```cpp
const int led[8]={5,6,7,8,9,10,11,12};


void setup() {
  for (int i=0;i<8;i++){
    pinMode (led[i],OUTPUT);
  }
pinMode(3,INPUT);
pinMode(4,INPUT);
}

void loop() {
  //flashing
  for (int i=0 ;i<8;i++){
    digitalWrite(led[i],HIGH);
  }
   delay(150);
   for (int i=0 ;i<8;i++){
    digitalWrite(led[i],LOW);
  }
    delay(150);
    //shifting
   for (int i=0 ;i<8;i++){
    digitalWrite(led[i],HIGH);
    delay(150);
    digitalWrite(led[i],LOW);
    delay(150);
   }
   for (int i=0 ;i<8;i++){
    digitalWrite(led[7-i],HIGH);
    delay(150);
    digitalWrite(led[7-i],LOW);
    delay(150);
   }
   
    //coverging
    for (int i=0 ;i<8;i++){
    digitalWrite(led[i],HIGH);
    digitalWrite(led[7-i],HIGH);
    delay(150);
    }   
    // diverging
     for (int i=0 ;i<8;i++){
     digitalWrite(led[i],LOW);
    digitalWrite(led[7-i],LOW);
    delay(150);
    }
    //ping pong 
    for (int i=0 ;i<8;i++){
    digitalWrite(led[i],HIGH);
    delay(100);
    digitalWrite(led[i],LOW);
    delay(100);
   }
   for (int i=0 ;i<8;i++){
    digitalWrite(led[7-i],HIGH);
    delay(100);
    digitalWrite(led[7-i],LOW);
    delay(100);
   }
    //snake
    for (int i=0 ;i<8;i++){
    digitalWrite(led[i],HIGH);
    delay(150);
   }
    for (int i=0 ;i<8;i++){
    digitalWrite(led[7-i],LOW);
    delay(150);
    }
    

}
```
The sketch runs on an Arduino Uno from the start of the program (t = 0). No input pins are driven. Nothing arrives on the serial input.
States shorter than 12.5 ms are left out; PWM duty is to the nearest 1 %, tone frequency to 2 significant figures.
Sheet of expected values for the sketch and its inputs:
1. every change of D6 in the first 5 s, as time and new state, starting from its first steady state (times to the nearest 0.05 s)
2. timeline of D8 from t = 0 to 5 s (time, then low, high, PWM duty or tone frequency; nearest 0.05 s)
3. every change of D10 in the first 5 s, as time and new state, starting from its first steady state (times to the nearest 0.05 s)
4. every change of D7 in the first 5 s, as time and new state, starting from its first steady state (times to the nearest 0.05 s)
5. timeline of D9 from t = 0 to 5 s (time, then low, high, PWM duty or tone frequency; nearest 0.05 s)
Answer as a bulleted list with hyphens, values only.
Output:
- 0 s high; 0.15 s low; 0.6 s high; 0.75 s low; 4.5 s high; 4.65 s low
- 0 s high; 0.15 s low; 1.2 s high; 1.35 s low; 3.9 s high; 4.05 s low
- 0 s high; 0.15 s low; 1.8 s high; 1.95 s low; 3.3 s high; 3.45 s low
- 0 s high; 0.15 s low; 0.9 s high; 1.05 s low; 4.2 s high; 4.35 s low
- 0 s high; 0.15 s low; 1.5 s high; 1.65 s low; 3.6 s high; 3.75 s low
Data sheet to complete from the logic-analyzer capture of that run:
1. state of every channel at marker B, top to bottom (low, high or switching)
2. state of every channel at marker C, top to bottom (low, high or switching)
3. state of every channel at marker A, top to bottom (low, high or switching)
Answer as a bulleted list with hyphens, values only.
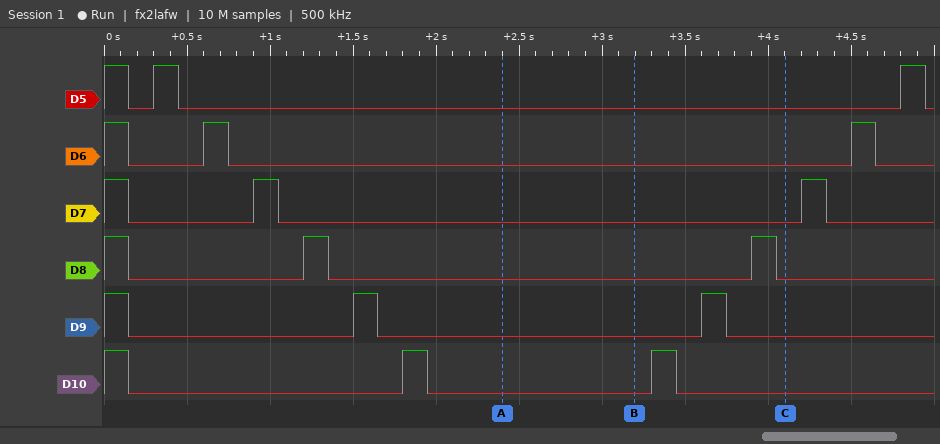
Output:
- D5 low, D6 low, D7 low, D8 low, D9 low, D10 low
- D5 low, D6 low, D7 low, D8 low, D9 low, D10 low
- D5 low, D6 low, D7 low, D8 low, D9 low, D10 low
